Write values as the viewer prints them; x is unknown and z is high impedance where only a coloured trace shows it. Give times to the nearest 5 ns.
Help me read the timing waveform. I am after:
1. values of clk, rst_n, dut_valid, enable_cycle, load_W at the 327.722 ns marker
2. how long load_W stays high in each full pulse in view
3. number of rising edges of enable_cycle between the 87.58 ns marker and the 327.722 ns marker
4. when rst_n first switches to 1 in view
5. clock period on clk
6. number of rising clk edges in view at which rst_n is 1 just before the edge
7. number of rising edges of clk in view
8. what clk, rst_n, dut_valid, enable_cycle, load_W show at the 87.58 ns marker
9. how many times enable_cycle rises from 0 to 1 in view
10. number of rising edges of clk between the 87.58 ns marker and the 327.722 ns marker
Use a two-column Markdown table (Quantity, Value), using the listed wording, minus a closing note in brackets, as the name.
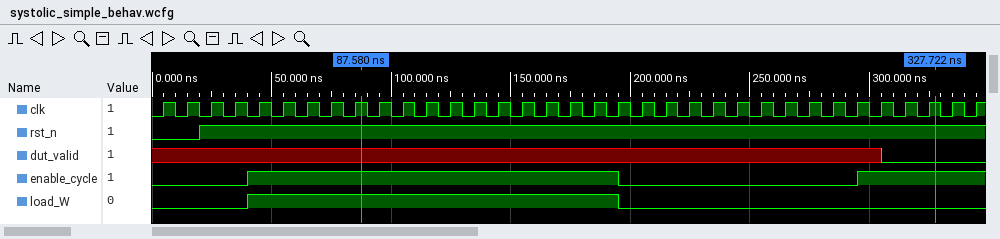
| Quantity | Value |
|---|---|
| values of clk, rst_n, dut_valid, enable_cycle, load_W at the 327.722 ns marker | clk=1, rst_n=1, dut_valid=0, enable_cycle=1, load_W=0 |
| how long load_W stays high in each full pulse in view | 155 ns |
| number of rising edges of enable_cycle between the 87.58 ns marker and the 327.722 ns marker | 1 |
| when rst_n first switches to 1 in view | 20 ns |
| clock period on clk | 10 ns |
| number of rising clk edges in view at which rst_n is 1 just before the edge | 33 |
| number of rising edges of clk in view | 35 |
| what clk, rst_n, dut_valid, enable_cycle, load_W show at the 87.58 ns marker | clk=1, rst_n=1, dut_valid=x, enable_cycle=1, load_W=1 |
| how many times enable_cycle rises from 0 to 1 in view | 2 |
| number of rising edges of clk between the 87.58 ns marker and the 327.722 ns marker | 24 |
